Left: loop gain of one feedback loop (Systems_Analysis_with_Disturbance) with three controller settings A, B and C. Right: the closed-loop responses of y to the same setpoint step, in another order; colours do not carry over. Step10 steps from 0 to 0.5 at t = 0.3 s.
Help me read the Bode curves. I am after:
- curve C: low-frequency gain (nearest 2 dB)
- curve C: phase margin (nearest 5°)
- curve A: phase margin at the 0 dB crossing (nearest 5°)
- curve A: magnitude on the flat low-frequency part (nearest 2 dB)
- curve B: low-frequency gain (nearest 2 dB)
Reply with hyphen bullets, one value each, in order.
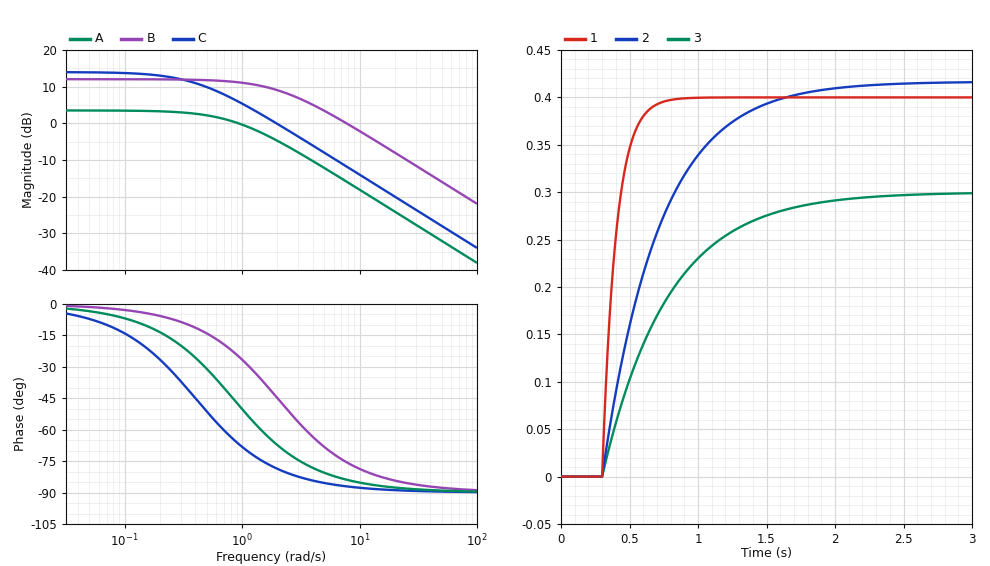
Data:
- 14 dB
- 100°
- 130°
- 4 dB
- 12 dB
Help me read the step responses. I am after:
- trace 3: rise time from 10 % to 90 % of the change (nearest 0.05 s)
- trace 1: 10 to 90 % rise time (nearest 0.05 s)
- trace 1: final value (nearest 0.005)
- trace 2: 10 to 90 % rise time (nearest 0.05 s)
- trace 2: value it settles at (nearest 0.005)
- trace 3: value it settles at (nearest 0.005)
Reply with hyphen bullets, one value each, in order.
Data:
- 1.05 s
- 0.20 s
- 0.400
- 0.90 s
- 0.415
- 0.300
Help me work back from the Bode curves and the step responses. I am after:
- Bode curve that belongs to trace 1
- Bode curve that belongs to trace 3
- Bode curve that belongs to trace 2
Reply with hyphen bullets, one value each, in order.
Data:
- B
- A
- C
